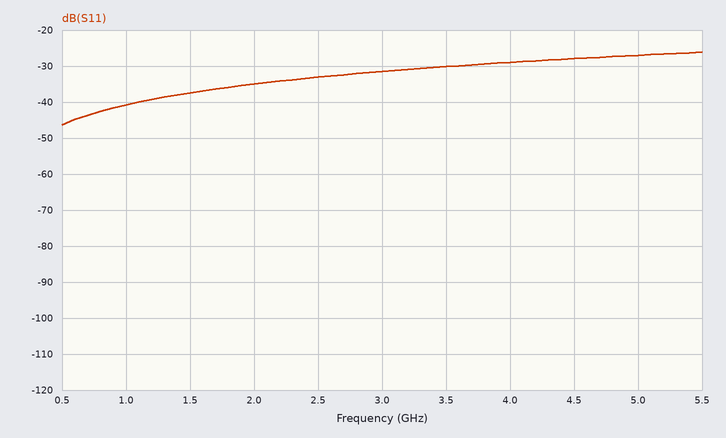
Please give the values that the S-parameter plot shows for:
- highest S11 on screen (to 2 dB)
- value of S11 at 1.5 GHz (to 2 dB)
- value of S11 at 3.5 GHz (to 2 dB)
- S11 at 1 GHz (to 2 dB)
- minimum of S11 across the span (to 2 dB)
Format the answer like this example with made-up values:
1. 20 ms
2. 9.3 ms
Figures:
1. -26 dB
2. -38 dB
3. -30 dB
4. -40 dB
5. -46 dB
